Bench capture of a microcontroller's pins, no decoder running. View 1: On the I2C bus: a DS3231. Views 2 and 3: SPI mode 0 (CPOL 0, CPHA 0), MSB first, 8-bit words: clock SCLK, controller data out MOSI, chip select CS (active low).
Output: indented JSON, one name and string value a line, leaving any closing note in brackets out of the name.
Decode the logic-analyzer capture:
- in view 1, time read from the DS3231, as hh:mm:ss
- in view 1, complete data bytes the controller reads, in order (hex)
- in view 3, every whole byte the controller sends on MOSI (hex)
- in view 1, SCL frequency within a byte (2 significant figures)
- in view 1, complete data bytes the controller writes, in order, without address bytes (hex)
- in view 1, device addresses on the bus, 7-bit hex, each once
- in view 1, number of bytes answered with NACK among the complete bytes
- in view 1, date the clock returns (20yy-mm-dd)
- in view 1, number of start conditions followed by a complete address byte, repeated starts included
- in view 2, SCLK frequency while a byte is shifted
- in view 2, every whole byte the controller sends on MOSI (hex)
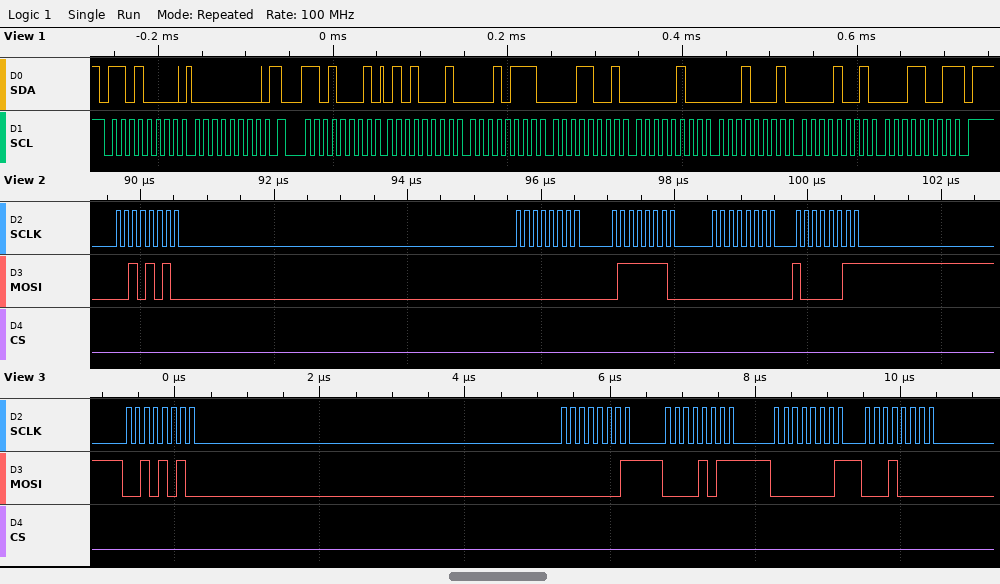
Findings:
{
  "in view 1, time read from the DS3231, as hh:mm:ss": "19:17:51",
  "in view 1, complete data bytes the controller reads, in order": "51 17 19 04 11 09 19",
  "in view 3, every whole byte the controller sends on MOSI": "2A 01 0B 01 10",
  "in view 1, SCL frequency within a byte": "100 kHz",
  "in view 1, complete data bytes the controller writes, in order, without address bytes": "00",
  "in view 1, device addresses on the bus, 7-bit hex, each once": "0x68",
  "in view 1, number of bytes answered with NACK among the complete bytes": "1",
  "in view 1, date the clock returns": "2019-09-11",
  "in view 1, number of start conditions followed by a complete address byte, repeated starts included": "2",
  "in view 2, SCLK frequency while a byte is shifted": "8 MHz",
  "in view 2, every whole byte the controller sends on MOSI": "0x2A 0x00 0x7E 0x00 0x83"
}
